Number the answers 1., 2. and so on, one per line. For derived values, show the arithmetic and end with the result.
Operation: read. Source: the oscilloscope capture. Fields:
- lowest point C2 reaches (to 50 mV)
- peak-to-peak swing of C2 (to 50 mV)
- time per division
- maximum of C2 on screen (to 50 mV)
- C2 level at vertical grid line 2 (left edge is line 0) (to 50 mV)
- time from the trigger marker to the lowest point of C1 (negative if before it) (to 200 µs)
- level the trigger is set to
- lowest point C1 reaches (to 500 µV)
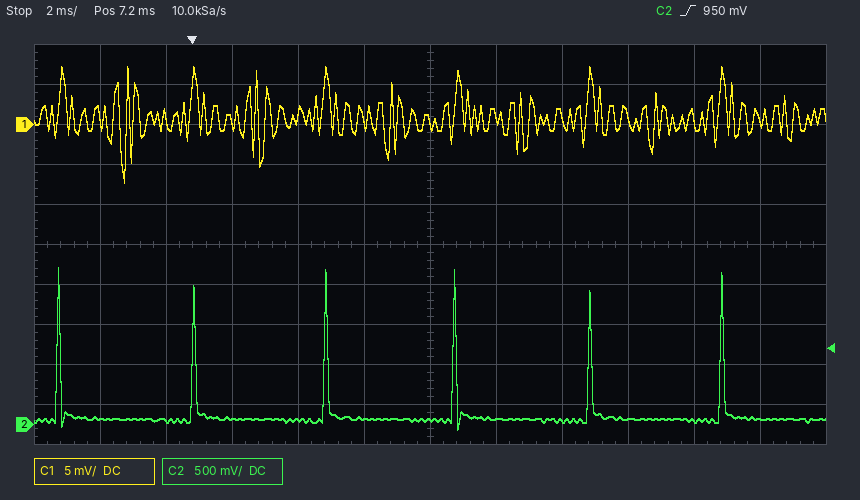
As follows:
1. -50 mV
2. 1.95 V − (-50 mV) = 2.00 V
3. 2 ms
4. 1.95 V
5. 50 mV
6. -2.0 ms
7. 950 mV
8. -7.0 mV
